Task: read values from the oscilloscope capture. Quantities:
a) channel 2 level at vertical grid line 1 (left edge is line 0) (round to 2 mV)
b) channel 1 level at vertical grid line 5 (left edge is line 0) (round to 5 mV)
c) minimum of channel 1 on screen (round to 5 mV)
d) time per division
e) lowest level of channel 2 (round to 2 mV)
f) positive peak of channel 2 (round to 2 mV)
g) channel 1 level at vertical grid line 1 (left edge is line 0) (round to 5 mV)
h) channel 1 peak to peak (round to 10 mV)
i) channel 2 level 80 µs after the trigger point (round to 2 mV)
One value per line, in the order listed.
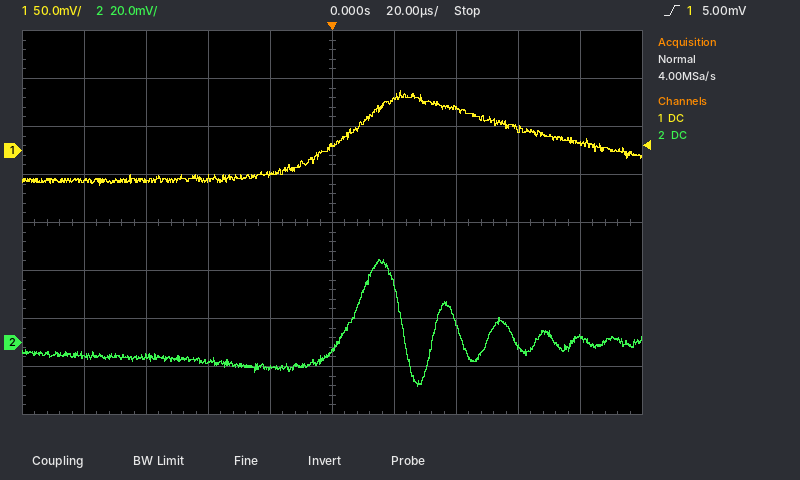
-6 mV
5 mV
-35 mV
20 µs
-18 mV
34 mV
-30 mV
100 mV
2 mV
